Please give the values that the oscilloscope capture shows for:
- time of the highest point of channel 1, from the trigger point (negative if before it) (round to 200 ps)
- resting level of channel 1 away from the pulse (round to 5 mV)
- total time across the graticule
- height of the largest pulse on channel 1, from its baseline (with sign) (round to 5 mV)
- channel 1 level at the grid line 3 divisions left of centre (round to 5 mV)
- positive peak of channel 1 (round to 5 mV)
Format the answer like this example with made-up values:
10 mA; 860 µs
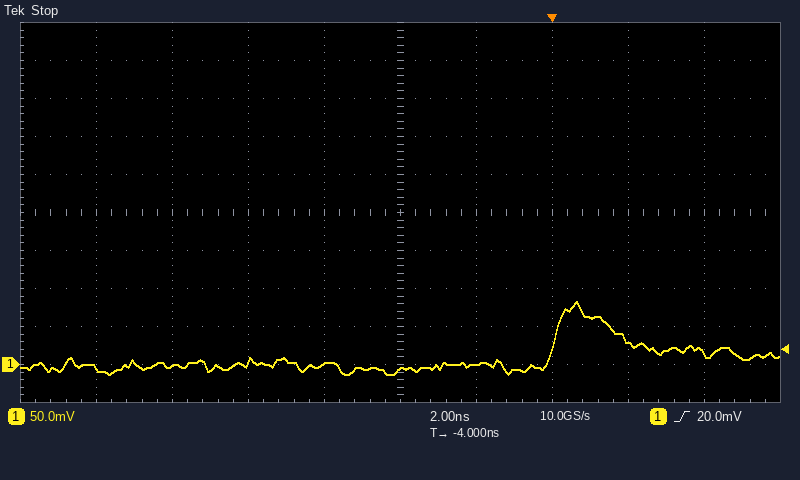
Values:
+600 ps; 0 mV; 20 ns; +85 mV; 0 mV; 85 mV
